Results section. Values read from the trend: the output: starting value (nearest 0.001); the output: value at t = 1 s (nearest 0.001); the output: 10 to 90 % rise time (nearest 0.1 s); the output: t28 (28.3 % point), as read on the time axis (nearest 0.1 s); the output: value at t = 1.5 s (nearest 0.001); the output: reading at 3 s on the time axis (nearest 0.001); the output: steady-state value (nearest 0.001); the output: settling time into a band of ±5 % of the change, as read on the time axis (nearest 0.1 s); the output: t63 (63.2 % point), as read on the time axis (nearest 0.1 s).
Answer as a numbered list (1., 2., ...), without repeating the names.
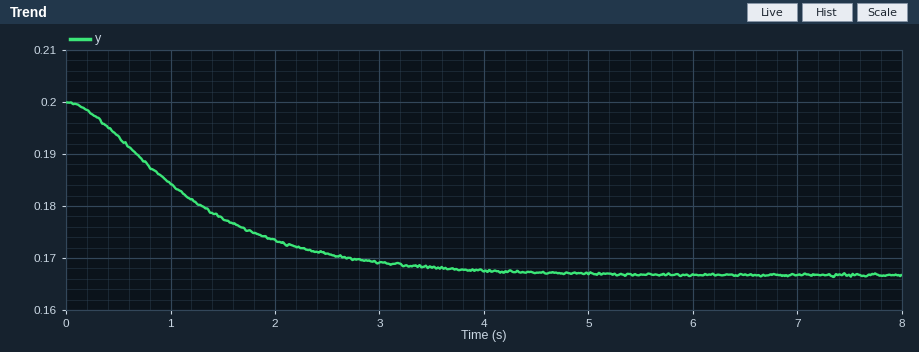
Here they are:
1. 0.200
2. 0.184
3. 2.4 s
4. 0.6 s
5. 0.178
6. 0.169
7. 0.167
8. 3.4 s
9. 1.4 s
